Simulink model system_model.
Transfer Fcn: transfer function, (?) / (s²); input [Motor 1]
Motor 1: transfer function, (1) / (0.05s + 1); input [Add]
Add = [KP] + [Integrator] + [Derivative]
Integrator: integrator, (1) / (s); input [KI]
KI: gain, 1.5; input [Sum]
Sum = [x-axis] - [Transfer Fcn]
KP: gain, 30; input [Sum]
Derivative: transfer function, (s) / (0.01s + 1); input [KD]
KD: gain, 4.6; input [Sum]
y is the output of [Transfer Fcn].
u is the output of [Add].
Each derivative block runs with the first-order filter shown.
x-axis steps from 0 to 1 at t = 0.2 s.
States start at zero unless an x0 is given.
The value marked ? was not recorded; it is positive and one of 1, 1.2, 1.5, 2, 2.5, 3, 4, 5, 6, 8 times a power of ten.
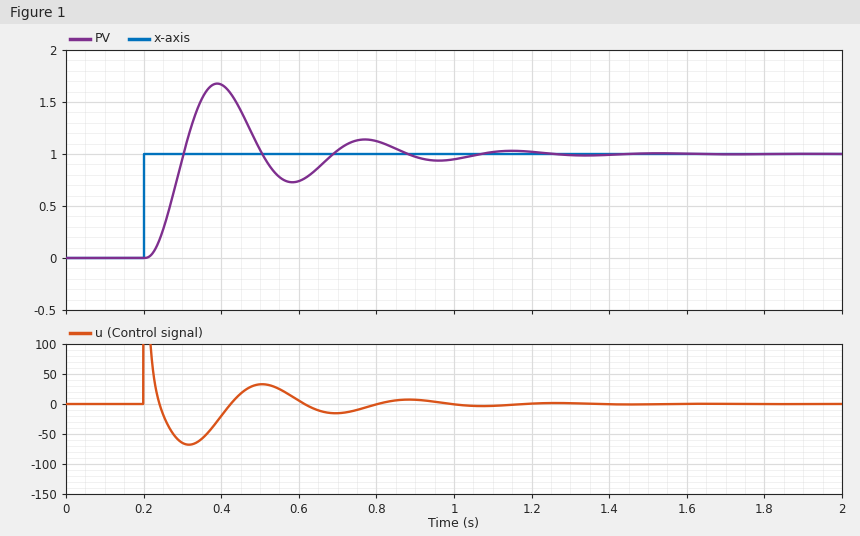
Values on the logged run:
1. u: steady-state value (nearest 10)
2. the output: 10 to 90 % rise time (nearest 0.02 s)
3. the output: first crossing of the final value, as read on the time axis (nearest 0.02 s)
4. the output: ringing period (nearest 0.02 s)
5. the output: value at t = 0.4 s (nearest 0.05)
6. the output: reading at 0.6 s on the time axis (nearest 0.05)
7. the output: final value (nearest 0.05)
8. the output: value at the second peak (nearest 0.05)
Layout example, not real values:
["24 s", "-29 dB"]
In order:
["0", "0.06 s", "0.30 s", "0.38 s", "1.65", "0.75", "1.00", "1.15"]
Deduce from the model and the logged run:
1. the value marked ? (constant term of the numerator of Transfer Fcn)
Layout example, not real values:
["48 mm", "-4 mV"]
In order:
["4"]
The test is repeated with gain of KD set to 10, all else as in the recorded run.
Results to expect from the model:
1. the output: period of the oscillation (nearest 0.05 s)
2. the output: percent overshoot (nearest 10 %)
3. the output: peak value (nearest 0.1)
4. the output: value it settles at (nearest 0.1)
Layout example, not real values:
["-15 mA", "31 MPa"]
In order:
["0.25 s", "70 %", "1.7", "1.0"]
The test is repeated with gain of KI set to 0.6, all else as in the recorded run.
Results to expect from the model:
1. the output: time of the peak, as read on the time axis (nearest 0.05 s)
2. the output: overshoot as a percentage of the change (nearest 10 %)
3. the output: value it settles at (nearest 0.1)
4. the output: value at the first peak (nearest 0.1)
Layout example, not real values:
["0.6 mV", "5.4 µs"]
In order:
["0.40 s", "70 %", "1.0", "1.7"]
